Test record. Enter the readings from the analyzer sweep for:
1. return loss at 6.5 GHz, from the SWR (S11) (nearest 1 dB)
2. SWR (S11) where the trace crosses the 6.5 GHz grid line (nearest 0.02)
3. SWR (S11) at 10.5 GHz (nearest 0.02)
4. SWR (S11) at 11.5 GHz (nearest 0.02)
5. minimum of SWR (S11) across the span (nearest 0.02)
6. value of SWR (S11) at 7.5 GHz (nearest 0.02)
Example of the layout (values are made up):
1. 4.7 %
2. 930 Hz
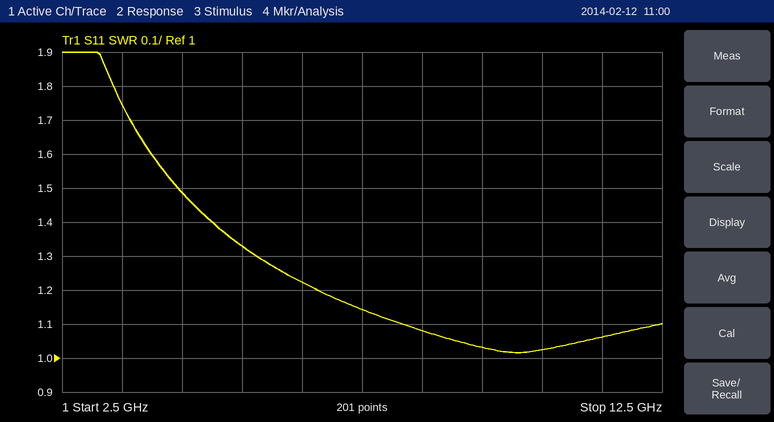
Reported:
1. 20 dB
2. 1.22
3. 1.02
4. 1.06
5. 1.02
6. 1.14
